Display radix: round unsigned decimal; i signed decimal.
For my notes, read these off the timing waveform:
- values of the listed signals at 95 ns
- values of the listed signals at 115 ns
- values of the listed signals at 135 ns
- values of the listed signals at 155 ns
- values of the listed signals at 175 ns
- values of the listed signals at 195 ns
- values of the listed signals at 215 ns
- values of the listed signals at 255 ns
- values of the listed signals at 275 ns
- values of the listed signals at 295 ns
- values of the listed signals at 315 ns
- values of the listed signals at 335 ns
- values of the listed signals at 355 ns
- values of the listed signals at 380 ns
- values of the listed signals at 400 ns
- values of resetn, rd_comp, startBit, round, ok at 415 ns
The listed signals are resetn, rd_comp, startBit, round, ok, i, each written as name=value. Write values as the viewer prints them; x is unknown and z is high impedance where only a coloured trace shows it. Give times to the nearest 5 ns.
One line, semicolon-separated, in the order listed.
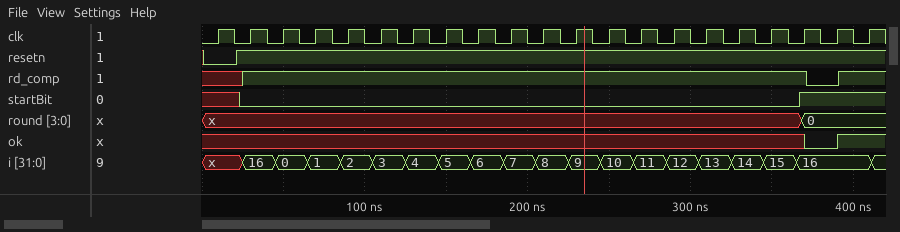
resetn=1, rd_comp=1, startBit=0, round=x, ok=x, i=2; resetn=1, rd_comp=1, startBit=0, round=x, ok=x, i=3; resetn=1, rd_comp=1, startBit=0, round=x, ok=x, i=4; resetn=1, rd_comp=1, startBit=0, round=x, ok=x, i=5; resetn=1, rd_comp=1, startBit=0, round=x, ok=x, i=6; resetn=1, rd_comp=1, startBit=0, round=x, ok=x, i=7; resetn=1, rd_comp=1, startBit=0, round=x, ok=x, i=8; resetn=1, rd_comp=1, startBit=0, round=x, ok=x, i=10; resetn=1, rd_comp=1, startBit=0, round=x, ok=x, i=11; resetn=1, rd_comp=1, startBit=0, round=x, ok=x, i=12; resetn=1, rd_comp=1, startBit=0, round=x, ok=x, i=13; resetn=1, rd_comp=1, startBit=0, round=x, ok=x, i=14; resetn=1, rd_comp=1, startBit=0, round=x, ok=x, i=15; resetn=1, rd_comp=0, startBit=1, round=0, ok=0, i=16; resetn=1, rd_comp=1, startBit=1, round=0, ok=1, i=16; resetn=1, rd_comp=1, startBit=1, round=0, ok=1
